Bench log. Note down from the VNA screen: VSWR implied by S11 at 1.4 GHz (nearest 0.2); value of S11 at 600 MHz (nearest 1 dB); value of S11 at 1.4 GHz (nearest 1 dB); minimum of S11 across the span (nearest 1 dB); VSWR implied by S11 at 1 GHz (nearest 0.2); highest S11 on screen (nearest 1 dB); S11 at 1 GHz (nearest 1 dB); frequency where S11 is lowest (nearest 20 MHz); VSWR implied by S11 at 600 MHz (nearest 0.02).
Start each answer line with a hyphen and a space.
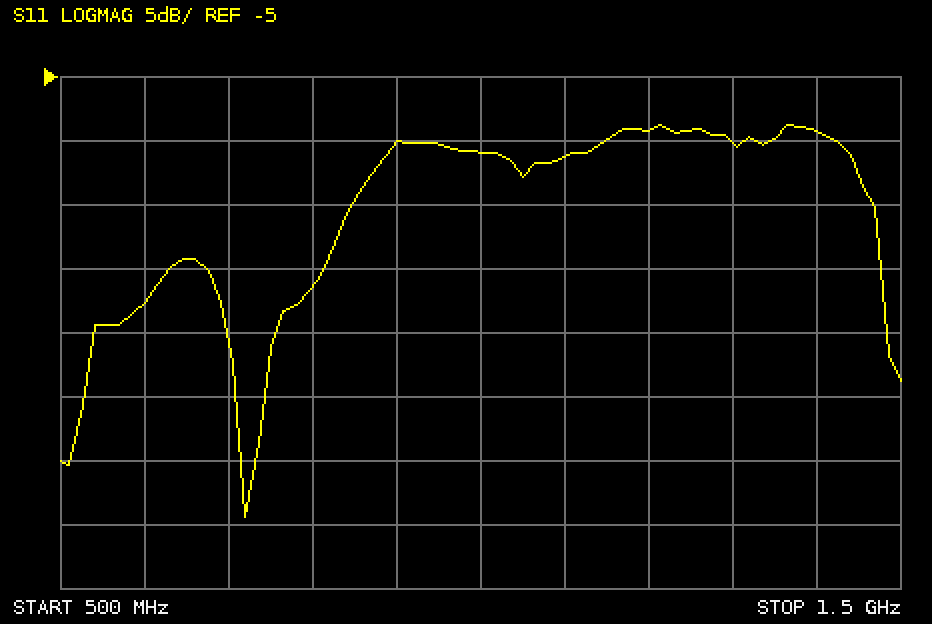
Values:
- 2.0
- -23 dB
- -9 dB
- -39 dB
- 1.8
- -9 dB
- -11 dB
- 720 MHz
- 1.16
